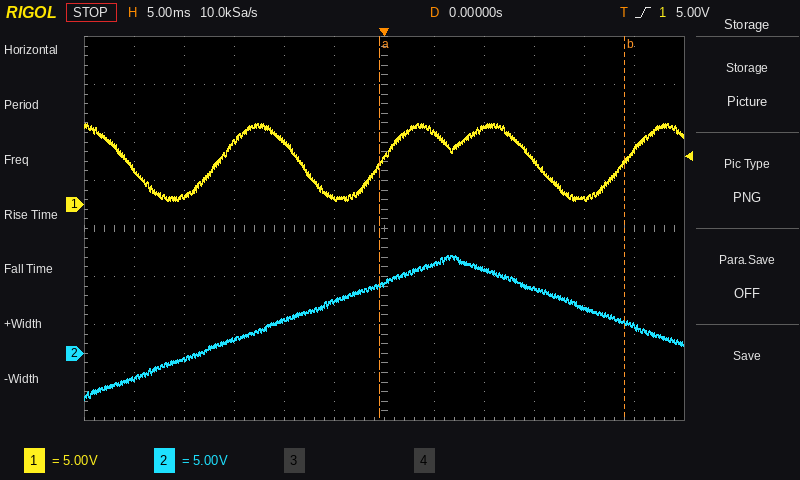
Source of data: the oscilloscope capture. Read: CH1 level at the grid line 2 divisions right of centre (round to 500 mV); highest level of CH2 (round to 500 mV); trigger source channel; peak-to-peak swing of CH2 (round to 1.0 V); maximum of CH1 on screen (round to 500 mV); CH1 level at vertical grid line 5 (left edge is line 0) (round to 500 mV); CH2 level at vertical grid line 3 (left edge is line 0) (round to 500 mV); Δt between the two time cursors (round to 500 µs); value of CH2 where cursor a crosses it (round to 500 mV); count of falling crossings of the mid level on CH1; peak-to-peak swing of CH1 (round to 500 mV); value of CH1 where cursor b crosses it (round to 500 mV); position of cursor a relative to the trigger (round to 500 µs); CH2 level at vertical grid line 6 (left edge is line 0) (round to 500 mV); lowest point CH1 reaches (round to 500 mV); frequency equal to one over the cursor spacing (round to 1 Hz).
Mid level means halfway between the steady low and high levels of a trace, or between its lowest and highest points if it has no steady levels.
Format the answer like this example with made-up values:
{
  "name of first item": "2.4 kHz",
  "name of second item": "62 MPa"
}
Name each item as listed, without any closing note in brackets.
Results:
{
  "CH1 level at the grid line 2 divisions right of centre": "8.0 V",
  "highest level of CH2": "10.0 V",
  "trigger source channel": "CH1",
  "peak-to-peak swing of CH2": "15.0 V",
  "maximum of CH1 on screen": "8.5 V",
  "CH1 level at vertical grid line 5 (left edge is line 0)": "500 mV",
  "CH2 level at vertical grid line 3 (left edge is line 0)": "1.5 V",
  "Δt between the two time cursors": "24.5 ms",
  "value of CH2 where cursor a crosses it": "7.0 V",
  "count of falling crossings of the mid level on CH1": "3",
  "peak-to-peak swing of CH1": "8.0 V",
  "value of CH1 where cursor b crosses it": "4.5 V",
  "position of cursor a relative to the trigger": "-500 µs",
  "CH2 level at vertical grid line 6 (left edge is line 0)": "7.5 V",
  "lowest point CH1 reaches": "500 mV",
  "frequency equal to one over the cursor spacing": "41 Hz"
}
